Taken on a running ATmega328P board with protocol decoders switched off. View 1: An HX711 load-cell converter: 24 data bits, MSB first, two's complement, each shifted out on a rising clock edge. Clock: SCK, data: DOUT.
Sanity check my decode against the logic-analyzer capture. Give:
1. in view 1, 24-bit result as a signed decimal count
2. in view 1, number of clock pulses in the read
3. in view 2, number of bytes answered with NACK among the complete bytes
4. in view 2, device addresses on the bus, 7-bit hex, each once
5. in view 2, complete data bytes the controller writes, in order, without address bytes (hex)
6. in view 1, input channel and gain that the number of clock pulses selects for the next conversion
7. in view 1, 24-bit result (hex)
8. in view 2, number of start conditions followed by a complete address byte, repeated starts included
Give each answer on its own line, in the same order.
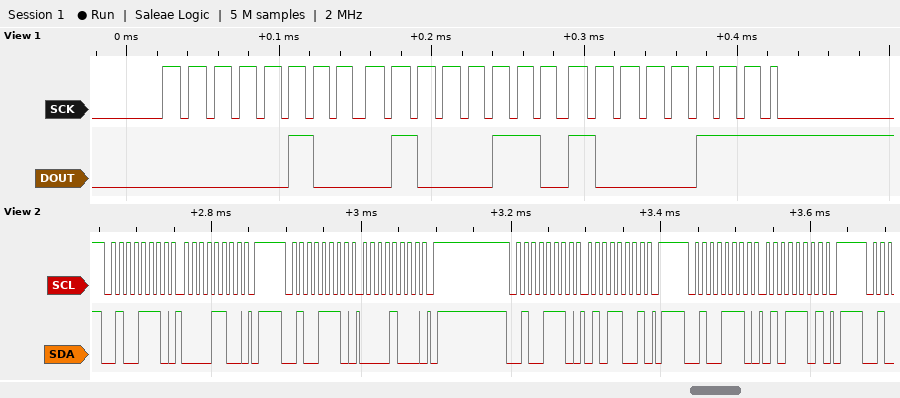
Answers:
280199
25
0
0x27
0C 08 59 5D
channel A, gain 128
0x044687
4
